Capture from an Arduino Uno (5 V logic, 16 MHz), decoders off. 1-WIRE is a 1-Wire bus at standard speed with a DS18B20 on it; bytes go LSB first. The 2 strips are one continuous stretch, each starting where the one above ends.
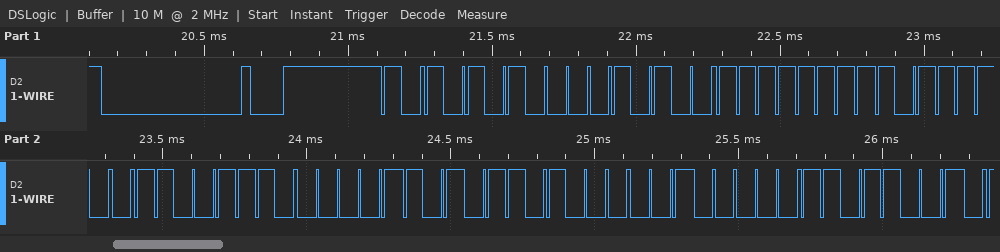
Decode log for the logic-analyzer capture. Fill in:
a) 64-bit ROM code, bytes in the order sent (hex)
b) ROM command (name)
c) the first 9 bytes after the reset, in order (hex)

28 FF 3D 73 B0 16 04 9B
Match ROM
55 28 FF 3D 73 B0 16 04 9B
